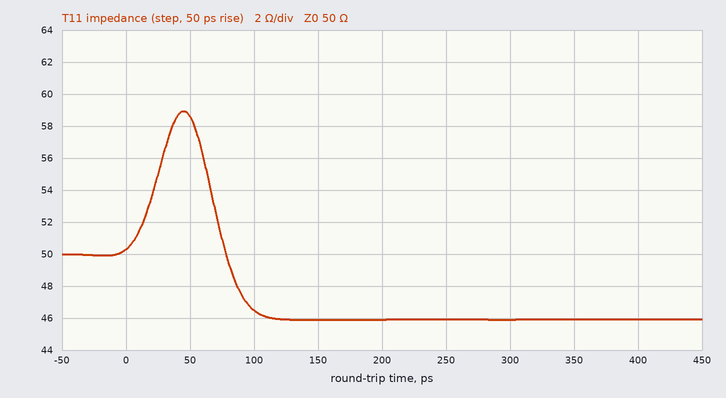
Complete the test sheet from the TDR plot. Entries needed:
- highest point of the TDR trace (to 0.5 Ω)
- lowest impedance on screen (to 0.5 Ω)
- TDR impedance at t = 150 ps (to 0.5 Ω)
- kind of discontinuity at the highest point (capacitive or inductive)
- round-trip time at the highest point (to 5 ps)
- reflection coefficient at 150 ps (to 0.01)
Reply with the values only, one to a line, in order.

59.0 Ω
46.0 Ω
46.0 Ω
inductive
45 ps
-0.04
